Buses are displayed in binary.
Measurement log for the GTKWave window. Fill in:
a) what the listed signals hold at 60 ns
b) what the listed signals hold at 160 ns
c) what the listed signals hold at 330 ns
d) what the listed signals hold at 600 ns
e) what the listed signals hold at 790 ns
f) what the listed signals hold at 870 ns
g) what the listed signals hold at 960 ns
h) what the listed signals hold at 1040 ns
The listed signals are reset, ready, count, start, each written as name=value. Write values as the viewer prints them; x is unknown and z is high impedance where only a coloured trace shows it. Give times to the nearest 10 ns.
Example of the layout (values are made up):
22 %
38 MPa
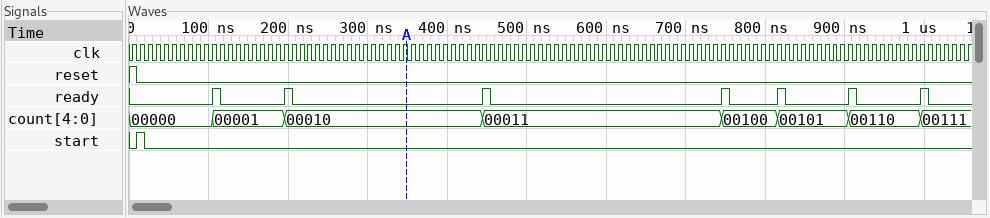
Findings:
reset=0, ready=0, count=00000, start=0
reset=0, ready=0, count=00001, start=0
reset=0, ready=0, count=00010, start=0
reset=0, ready=0, count=00011, start=0
reset=0, ready=0, count=00100, start=0
reset=0, ready=0, count=00101, start=0
reset=0, ready=0, count=00110, start=0
reset=0, ready=0, count=00111, start=0
